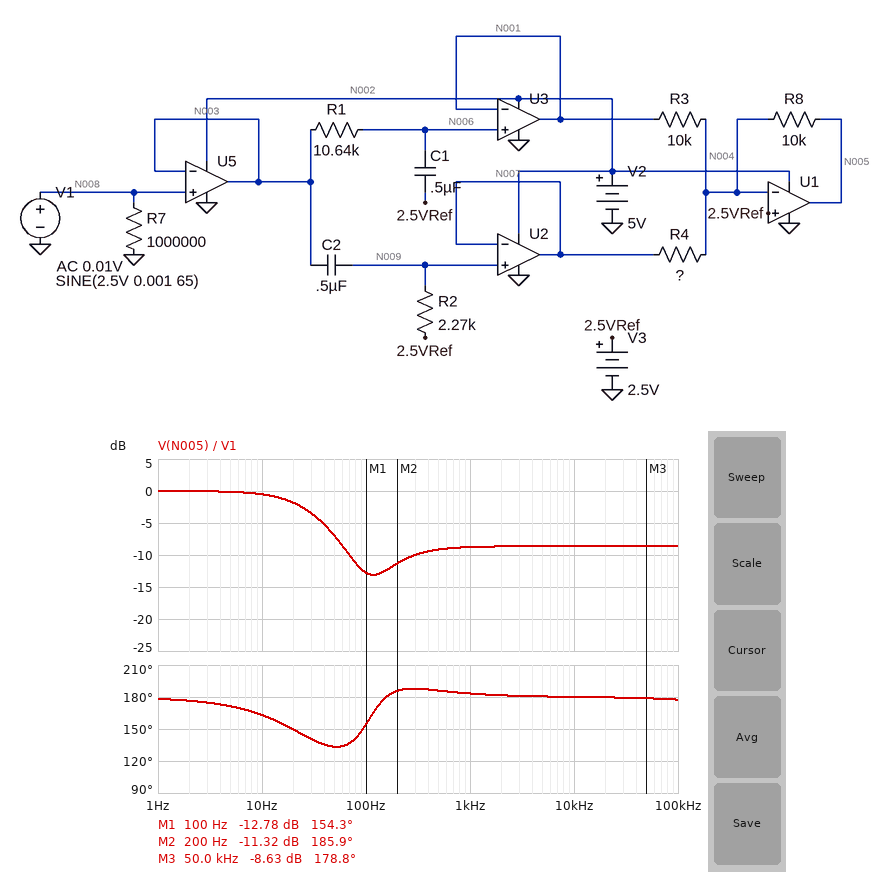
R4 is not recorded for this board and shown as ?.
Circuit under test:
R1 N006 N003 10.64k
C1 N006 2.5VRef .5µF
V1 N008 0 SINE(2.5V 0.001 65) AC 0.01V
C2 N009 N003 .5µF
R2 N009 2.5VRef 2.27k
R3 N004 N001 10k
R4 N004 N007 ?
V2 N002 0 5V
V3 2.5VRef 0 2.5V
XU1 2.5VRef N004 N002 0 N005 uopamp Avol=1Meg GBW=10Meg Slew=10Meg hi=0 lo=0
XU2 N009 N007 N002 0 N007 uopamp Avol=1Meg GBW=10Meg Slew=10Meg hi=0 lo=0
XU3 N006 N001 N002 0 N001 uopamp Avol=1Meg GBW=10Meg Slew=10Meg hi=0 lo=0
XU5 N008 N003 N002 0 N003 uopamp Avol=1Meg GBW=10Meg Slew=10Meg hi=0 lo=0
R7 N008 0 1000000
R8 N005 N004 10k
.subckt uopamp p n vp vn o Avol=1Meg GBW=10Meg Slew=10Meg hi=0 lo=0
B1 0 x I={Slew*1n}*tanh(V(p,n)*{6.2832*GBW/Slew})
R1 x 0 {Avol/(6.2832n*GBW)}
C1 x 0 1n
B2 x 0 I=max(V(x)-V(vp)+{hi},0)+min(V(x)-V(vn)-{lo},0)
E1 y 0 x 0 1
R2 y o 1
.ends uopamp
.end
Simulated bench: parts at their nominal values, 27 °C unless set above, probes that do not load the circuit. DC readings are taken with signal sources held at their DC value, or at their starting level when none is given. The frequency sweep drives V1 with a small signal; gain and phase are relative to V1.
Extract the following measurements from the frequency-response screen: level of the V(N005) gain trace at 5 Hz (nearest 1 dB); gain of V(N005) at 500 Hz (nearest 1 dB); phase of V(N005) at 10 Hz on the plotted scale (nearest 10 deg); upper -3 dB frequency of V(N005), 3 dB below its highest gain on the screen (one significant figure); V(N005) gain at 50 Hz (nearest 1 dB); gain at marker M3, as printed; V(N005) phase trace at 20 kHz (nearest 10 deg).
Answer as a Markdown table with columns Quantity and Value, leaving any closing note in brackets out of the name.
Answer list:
| Quantity | Value |
|---|---|
| level of the V(N005) gain trace at 5 Hz | 0 dB |
| gain of V(N005) at 500 Hz | -9 dB |
| phase of V(N005) at 10 Hz on the plotted scale | 160 deg |
| upper -3 dB frequency of V(N005), 3 dB below its highest gain on the screen | 30 Hz |
| V(N005) gain at 50 Hz | -7 dB |
| gain at marker M3, as printed | -8.63 dB |
| V(N005) phase trace at 20 kHz | 180 deg |
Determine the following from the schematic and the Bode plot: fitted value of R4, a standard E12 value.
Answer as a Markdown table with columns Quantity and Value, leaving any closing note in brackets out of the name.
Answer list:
| Quantity | Value |
|---|---|
| fitted value of R4, a standard E12 value | 27 kΩ |
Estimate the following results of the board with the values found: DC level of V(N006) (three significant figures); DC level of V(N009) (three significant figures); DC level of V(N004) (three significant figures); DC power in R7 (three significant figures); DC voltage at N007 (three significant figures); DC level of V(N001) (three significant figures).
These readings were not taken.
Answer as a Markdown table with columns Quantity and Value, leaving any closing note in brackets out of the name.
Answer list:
| Quantity | Value |
|---|---|
| DC level of V(N006) | 2.50 V |
| DC level of V(N009) | 2.50 V |
| DC level of V(N004) | 2.50 V |
| DC power in R7 | 6.25 µW |
| DC voltage at N007 | 2.50 V |
| DC level of V(N001) | 2.50 V |
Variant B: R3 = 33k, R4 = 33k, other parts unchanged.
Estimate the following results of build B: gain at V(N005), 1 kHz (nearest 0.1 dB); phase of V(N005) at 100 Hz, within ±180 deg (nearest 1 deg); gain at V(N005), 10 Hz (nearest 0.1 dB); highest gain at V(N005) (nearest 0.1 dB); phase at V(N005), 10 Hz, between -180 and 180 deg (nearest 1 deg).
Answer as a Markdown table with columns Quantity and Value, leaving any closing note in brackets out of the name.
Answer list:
| Quantity | Value |
|---|---|
| gain at V(N005), 1 kHz | -10.5 dB |
| phase of V(N005) at 100 Hz, within ±180 deg | -155 deg |
| gain at V(N005), 10 Hz | -11.0 dB |
| highest gain at V(N005) | -10.4 dB |
| phase at V(N005), 10 Hz, between -180 and 180 deg | 166 deg |
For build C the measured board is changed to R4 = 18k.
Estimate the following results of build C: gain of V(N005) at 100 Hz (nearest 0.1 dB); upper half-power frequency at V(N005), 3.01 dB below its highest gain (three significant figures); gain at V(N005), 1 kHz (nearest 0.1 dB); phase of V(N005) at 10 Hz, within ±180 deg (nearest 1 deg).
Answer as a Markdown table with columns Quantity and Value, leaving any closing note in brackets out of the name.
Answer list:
| Quantity | Value |
|---|---|
| gain of V(N005) at 100 Hz | -11.4 dB |
| upper half-power frequency at V(N005), 3.01 dB below its highest gain | 26.1 Hz |
| gain at V(N005), 1 kHz | -5.2 dB |
| phase of V(N005) at 10 Hz, within ±180 deg | 164 deg |
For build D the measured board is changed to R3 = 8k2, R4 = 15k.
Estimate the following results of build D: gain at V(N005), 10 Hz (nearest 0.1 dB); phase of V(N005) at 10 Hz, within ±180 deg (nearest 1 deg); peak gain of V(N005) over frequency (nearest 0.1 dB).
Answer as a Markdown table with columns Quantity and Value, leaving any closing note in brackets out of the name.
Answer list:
| Quantity | Value |
|---|---|
| gain at V(N005), 10 Hz | 1.2 dB |
| phase of V(N005) at 10 Hz, within ±180 deg | 164 deg |
| peak gain of V(N005) over frequency | 1.7 dB |
